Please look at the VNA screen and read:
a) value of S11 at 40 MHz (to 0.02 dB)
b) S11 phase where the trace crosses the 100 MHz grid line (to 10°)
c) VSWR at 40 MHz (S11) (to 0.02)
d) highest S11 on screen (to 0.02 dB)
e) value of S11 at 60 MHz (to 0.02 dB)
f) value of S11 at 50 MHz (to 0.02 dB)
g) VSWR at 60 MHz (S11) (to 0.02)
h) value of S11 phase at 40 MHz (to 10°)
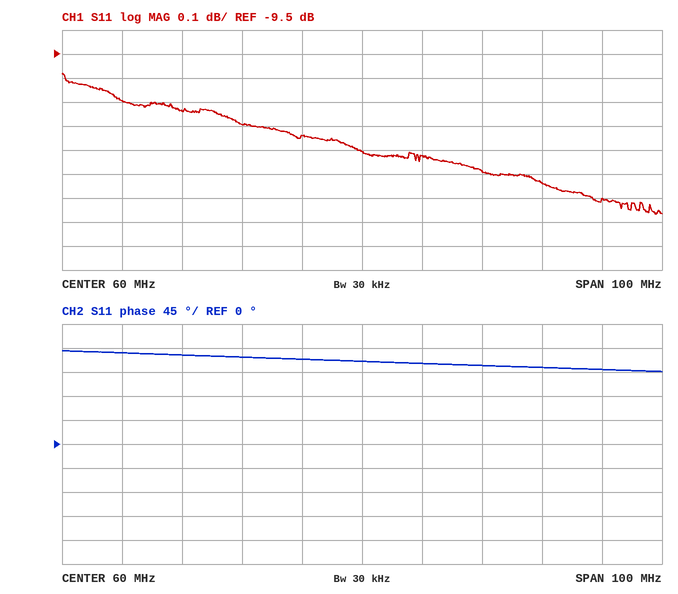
-9.80 dB
140°
1.96
-9.58 dB
-9.90 dB
-9.84 dB
1.94
160°
